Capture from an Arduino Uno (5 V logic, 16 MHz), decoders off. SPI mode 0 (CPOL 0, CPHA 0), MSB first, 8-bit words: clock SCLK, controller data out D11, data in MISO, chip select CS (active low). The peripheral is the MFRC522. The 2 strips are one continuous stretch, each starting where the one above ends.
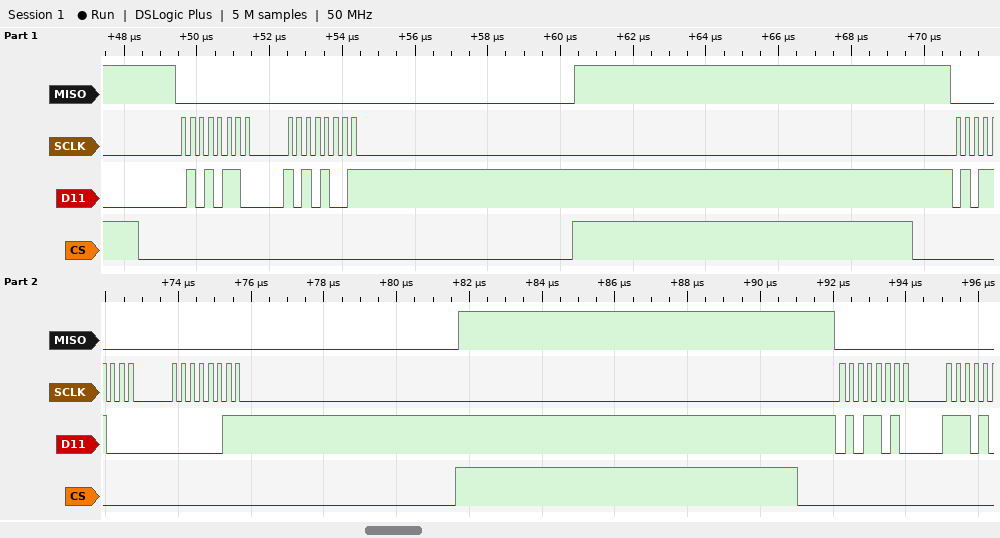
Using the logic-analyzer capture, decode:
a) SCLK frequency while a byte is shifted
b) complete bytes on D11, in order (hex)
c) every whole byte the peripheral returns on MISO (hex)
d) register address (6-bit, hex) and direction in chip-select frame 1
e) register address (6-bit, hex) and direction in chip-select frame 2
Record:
4 MHz
0x56 0xA9 0x58 0x03 0x5A
0x00 0x00 0x00 0x00 0x00
0x2B write
0x2C write
